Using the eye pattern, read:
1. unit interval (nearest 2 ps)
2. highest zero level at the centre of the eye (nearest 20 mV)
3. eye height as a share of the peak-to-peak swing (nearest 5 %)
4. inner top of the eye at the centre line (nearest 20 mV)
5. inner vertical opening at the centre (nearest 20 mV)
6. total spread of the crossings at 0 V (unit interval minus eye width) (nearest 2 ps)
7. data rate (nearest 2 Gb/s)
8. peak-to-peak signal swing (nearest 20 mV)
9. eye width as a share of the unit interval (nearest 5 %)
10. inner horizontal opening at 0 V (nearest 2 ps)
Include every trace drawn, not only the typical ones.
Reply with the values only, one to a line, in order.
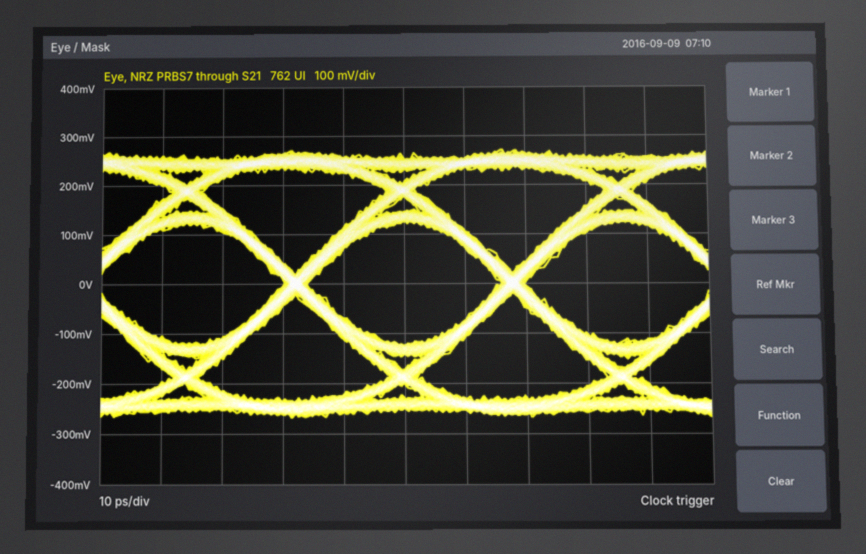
36 ps
-120 mV
45 %
120 mV
240 mV
4 ps
28 Gb/s
540 mV
90 %
32 ps
